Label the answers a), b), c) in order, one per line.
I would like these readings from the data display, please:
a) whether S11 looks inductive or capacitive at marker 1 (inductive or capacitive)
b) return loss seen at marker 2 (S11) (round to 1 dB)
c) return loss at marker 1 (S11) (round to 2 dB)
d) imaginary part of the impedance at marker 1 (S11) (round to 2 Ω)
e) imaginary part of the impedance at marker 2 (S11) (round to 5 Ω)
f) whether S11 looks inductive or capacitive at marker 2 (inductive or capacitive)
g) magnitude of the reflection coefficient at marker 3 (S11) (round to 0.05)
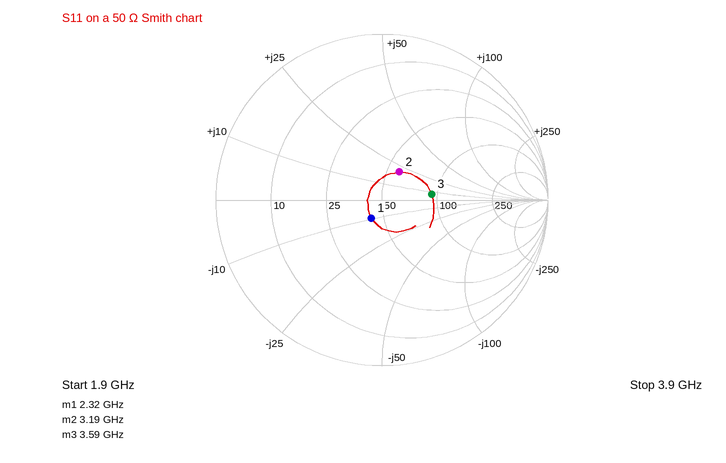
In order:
a) capacitive
b) 14 dB
c) 18 dB
d) -10 Ω
e) +20 Ω
f) inductive
g) 0.30
